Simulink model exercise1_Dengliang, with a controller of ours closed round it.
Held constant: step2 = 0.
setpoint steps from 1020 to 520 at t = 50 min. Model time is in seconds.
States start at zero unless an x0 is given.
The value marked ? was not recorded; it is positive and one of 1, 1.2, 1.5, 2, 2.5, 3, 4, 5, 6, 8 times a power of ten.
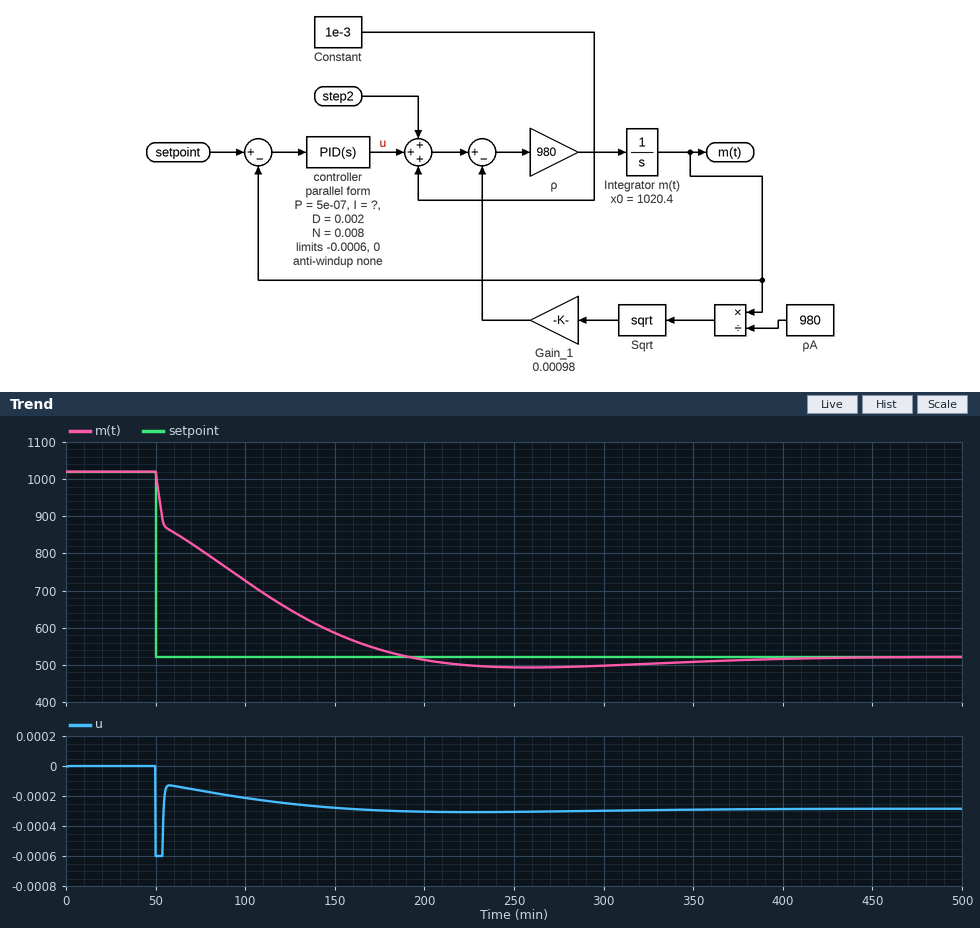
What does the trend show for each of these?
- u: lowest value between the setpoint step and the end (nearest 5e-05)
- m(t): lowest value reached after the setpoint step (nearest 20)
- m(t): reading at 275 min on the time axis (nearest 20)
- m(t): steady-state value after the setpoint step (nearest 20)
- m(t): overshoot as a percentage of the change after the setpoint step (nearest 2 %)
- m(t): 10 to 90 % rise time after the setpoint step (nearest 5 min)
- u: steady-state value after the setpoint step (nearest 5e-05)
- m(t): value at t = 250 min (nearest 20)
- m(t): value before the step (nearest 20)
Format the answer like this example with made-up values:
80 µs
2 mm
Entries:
-0.00060
500
500
520
6 %
105 min
-0.00030
500
1020
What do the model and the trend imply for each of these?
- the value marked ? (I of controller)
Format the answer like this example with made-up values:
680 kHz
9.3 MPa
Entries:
2.5e-10
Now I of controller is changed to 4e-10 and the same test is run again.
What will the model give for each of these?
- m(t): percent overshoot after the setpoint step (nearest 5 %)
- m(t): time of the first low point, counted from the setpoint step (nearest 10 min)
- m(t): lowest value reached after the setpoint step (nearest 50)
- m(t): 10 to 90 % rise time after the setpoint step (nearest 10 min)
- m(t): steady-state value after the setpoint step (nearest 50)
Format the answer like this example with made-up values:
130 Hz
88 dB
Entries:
10 %
150 min
450
80 min
500
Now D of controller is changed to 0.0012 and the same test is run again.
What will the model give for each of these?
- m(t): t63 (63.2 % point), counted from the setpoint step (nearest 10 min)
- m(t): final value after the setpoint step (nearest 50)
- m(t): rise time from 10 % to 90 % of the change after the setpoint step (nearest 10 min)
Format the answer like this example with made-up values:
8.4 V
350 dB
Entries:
50 min
500
100 min
